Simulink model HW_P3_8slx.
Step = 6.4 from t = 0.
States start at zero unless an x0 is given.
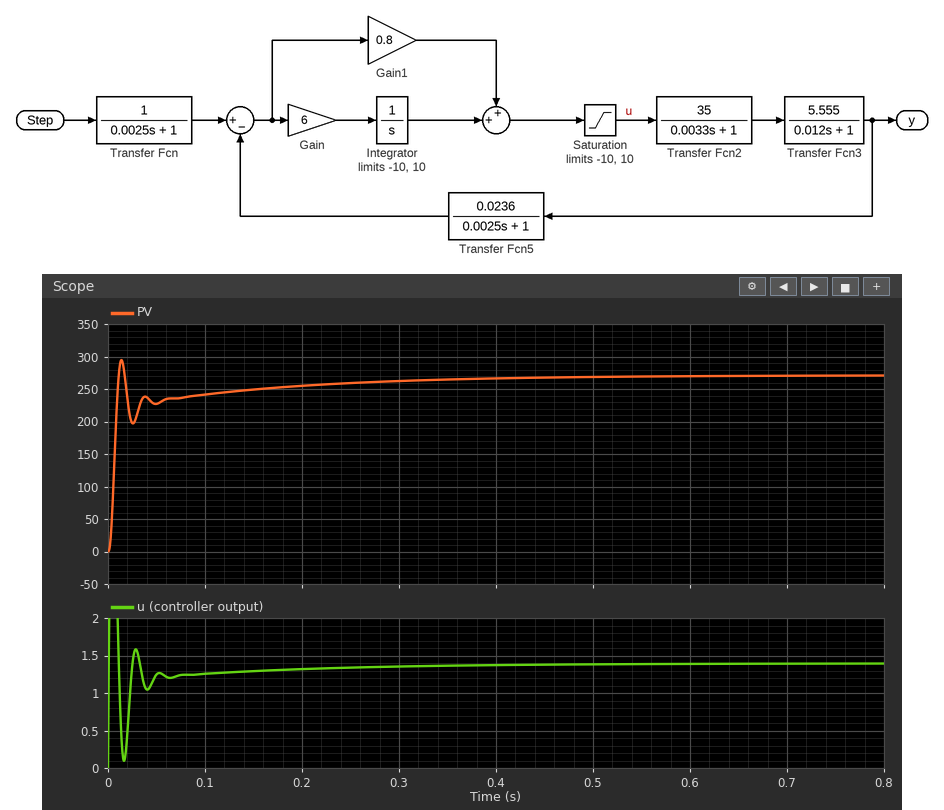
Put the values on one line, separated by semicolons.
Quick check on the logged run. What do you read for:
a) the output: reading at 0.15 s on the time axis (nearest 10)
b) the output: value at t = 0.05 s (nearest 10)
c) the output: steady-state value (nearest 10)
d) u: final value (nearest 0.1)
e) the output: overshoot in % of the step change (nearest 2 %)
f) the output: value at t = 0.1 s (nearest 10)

250; 230; 270; 1.4; 8 %; 240
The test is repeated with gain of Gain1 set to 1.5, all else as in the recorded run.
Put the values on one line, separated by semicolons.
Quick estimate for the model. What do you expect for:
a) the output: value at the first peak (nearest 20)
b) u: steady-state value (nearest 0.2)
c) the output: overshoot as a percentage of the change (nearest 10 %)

380; 1.4; 40 %
